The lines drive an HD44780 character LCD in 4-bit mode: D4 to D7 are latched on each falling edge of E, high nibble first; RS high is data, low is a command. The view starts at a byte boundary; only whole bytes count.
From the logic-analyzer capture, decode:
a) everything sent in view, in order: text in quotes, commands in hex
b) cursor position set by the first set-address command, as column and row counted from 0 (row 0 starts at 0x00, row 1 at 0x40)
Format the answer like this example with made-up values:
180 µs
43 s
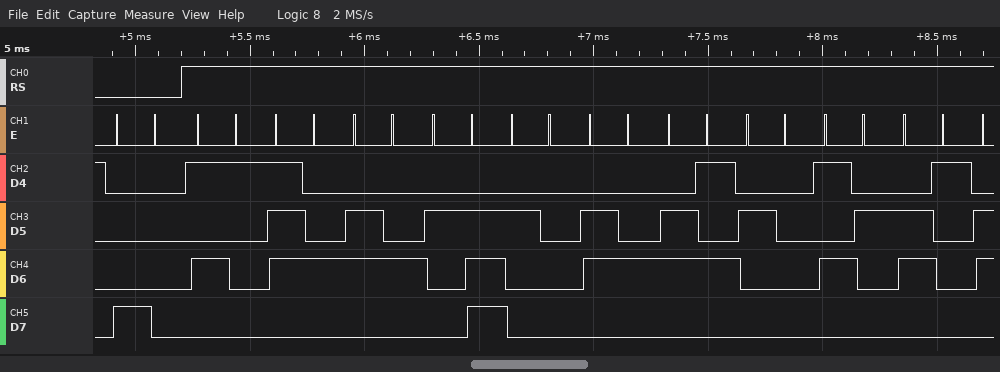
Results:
0x80 "Qtd. de Ra"
column 0, row 0
